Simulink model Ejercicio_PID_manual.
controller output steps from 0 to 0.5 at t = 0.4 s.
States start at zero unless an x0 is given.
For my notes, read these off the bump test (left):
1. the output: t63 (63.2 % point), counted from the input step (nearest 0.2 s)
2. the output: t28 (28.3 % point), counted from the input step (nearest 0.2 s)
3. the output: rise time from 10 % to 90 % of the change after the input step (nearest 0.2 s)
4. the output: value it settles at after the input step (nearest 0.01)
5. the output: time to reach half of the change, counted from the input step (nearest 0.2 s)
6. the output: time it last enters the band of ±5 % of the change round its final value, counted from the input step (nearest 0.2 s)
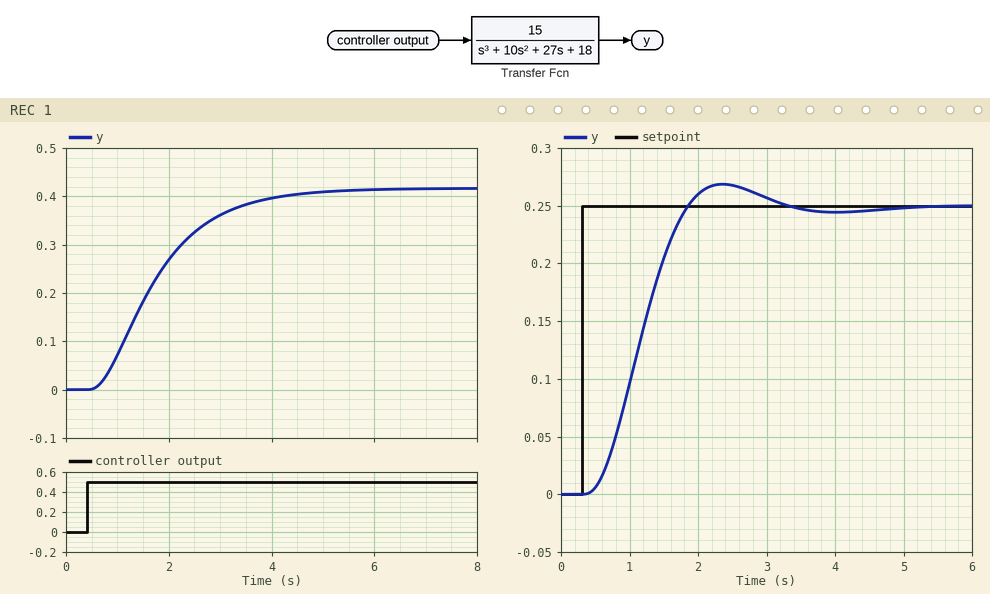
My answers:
1.6 s
0.8 s
2.4 s
0.42
1.2 s
3.6 s
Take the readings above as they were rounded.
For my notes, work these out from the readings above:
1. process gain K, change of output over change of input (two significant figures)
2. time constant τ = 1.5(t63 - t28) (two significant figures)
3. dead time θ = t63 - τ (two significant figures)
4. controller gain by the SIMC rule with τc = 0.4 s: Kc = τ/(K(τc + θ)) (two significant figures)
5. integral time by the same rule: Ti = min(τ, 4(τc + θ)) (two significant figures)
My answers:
0.84
1.2 s
0.40 s
1.8
1.2 s
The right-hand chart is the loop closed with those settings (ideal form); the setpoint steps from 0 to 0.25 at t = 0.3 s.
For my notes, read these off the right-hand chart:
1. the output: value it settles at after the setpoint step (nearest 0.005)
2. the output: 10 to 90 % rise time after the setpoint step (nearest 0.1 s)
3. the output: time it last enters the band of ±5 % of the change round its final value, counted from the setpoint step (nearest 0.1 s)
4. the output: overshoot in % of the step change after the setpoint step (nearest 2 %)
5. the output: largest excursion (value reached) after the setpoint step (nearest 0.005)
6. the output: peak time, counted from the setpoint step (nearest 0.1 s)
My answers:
0.250
1.0 s
2.5 s
8 %
0.270
2.1 s
